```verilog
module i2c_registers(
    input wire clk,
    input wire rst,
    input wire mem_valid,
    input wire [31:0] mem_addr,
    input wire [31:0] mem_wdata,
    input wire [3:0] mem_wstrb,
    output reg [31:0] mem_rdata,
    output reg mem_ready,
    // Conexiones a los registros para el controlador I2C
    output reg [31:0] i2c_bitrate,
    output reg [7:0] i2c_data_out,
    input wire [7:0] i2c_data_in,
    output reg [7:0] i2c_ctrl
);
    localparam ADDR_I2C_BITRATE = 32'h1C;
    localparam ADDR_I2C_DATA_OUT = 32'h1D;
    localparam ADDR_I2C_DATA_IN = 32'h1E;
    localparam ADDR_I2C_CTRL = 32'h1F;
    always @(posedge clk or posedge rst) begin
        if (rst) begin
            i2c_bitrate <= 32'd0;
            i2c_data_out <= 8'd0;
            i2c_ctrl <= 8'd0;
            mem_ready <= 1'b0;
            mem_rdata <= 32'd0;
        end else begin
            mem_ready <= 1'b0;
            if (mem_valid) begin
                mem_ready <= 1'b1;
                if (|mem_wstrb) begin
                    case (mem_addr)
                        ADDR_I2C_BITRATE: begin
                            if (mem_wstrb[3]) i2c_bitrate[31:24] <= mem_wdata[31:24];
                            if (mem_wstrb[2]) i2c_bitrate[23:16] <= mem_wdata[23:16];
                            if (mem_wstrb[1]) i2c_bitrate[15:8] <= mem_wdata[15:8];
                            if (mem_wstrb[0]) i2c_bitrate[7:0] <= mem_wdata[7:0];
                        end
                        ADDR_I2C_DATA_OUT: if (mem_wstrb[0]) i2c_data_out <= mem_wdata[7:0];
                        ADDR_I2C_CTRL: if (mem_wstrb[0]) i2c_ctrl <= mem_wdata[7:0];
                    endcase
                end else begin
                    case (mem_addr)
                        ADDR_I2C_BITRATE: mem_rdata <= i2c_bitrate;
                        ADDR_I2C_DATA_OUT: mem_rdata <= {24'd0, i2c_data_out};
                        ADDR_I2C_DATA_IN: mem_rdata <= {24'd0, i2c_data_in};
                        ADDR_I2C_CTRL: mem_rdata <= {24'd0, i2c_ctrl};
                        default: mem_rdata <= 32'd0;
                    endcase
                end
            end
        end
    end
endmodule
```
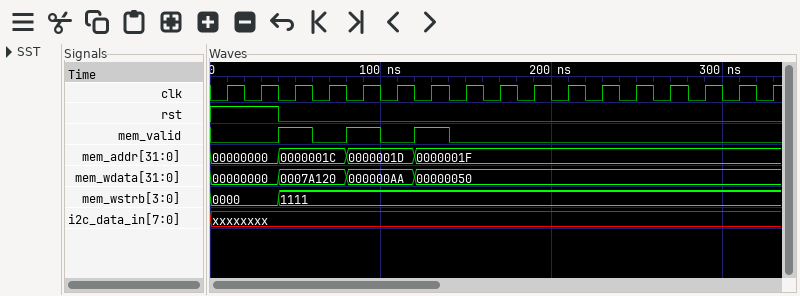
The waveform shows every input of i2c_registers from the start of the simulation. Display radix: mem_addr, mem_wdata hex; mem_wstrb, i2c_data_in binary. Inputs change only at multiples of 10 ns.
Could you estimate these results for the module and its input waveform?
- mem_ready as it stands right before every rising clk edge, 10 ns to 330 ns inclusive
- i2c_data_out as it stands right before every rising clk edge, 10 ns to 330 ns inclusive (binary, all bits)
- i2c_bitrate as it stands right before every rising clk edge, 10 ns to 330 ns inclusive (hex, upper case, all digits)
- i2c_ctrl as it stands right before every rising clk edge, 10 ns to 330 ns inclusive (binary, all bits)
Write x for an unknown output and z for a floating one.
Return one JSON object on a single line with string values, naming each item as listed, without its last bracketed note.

{"mem_ready as it stands right before every rising clk edge, 10 ns to 330 ns inclusive": "0 0 0 1 0 1 0 1 0 0 0 0 0 0 0 0 0", "i2c_data_out as it stands right before every rising clk edge, 10 ns to 330 ns inclusive": "00000000, 00000000, 00000000, 00000000, 00000000, 10101010, 10101010, 10101010, 10101010, 10101010, 10101010, 10101010, 10101010, 10101010, 10101010, 10101010, 10101010", "i2c_bitrate as it stands right before every rising clk edge, 10 ns to 330 ns inclusive": "00000000, 00000000, 00000000, 0007A120, 0007A120, 0007A120, 0007A120, 0007A120, 0007A120, 0007A120, 0007A120, 0007A120, 0007A120, 0007A120, 0007A120, 0007A120, 0007A120", "i2c_ctrl as it stands right before every rising clk edge, 10 ns to 330 ns inclusive": "00000000, 00000000, 00000000, 00000000, 00000000, 00000000, 00000000, 01010000, 01010000, 01010000, 01010000, 01010000, 01010000, 01010000, 01010000, 01010000, 01010000"}
